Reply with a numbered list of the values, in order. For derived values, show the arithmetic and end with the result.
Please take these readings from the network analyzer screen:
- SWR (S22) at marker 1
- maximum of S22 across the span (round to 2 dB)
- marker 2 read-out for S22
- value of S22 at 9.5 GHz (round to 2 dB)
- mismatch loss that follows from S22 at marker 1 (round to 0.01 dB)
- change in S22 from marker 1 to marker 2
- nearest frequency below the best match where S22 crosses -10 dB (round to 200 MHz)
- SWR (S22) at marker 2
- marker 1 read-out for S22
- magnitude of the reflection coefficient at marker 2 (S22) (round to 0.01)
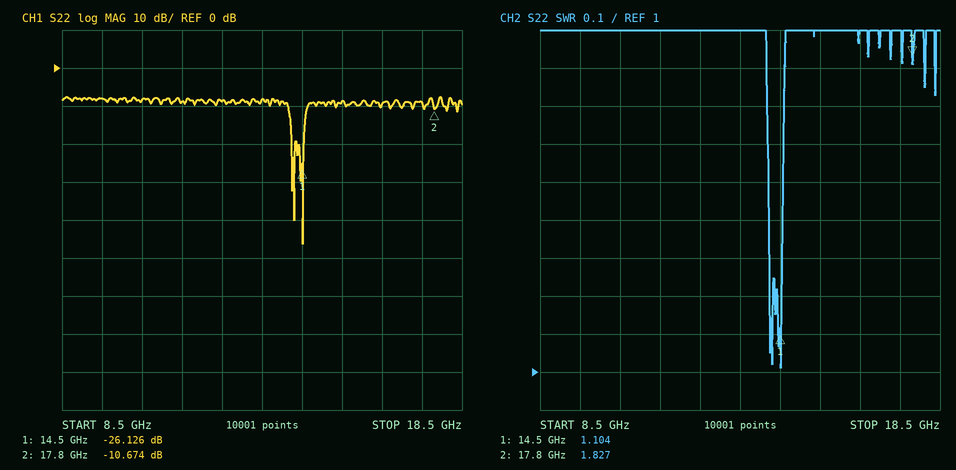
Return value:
1. 1.104
2. -8 dB
3. -10.674 dB
4. -8 dB
5. −10 log10(1 − 10^(-26.126/10)) ≈ 0.01 dB
6. -10.674 − (-26.126) = 15.452 dB
7. 14.2 GHz
8. 1.827
9. -26.126 dB
10. 10^(-10.674/20) ≈ 0.29
